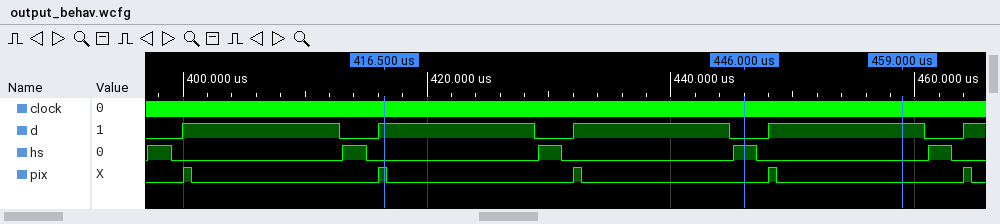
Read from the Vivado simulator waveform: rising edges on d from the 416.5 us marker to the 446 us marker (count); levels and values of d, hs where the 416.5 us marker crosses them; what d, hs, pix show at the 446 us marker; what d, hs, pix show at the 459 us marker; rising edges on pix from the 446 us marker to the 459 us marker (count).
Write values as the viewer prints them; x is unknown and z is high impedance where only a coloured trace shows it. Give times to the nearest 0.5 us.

1
d=1, hs=0
d=0, hs=1, pix=0
d=1, hs=0, pix=0
1
